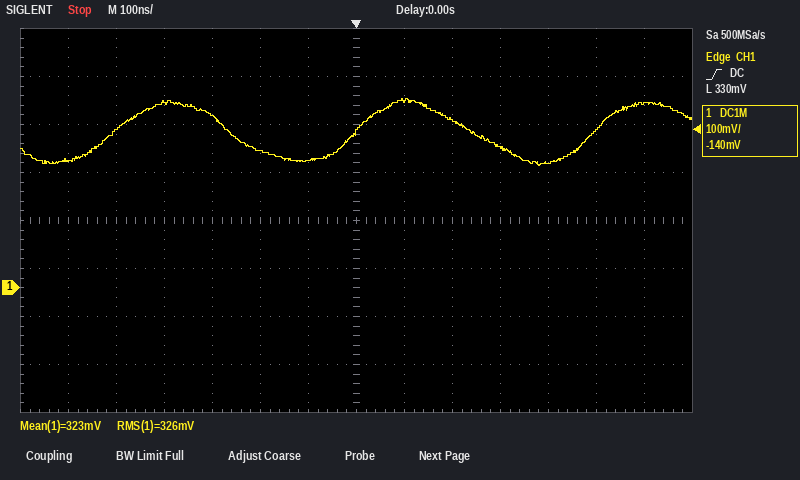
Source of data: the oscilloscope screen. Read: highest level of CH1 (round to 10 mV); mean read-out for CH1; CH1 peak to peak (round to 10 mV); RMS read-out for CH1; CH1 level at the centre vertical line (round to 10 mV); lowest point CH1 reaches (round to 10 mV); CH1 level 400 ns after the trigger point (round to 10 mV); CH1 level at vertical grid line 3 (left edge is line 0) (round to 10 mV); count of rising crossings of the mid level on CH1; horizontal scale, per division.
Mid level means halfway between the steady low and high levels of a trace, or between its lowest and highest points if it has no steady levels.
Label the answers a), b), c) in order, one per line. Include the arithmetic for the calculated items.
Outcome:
a) 390 mV
b) 323 mV
c) 390 mV − (250 mV) = 140 mV
d) 326 mV
e) 330 mV
f) 250 mV
g) 260 mV
h) 390 mV
i) 3
j) 100 ns
